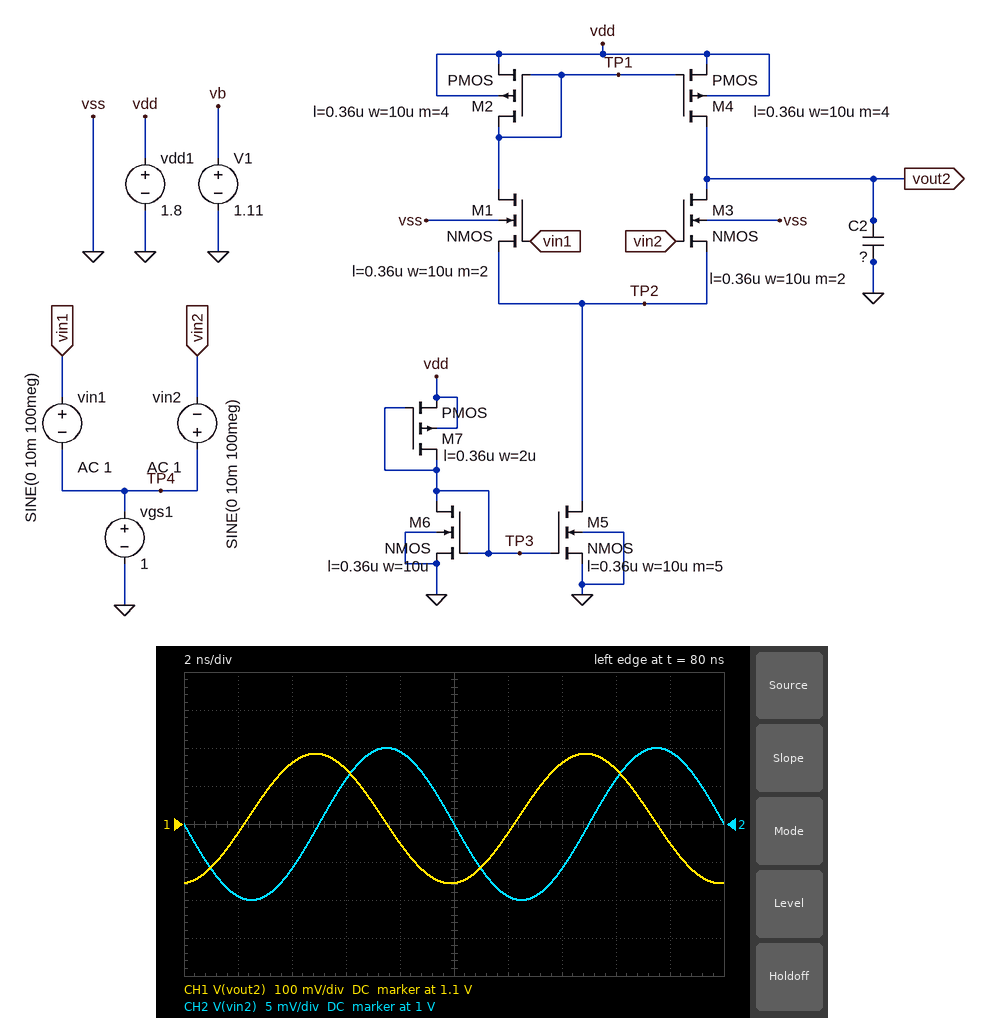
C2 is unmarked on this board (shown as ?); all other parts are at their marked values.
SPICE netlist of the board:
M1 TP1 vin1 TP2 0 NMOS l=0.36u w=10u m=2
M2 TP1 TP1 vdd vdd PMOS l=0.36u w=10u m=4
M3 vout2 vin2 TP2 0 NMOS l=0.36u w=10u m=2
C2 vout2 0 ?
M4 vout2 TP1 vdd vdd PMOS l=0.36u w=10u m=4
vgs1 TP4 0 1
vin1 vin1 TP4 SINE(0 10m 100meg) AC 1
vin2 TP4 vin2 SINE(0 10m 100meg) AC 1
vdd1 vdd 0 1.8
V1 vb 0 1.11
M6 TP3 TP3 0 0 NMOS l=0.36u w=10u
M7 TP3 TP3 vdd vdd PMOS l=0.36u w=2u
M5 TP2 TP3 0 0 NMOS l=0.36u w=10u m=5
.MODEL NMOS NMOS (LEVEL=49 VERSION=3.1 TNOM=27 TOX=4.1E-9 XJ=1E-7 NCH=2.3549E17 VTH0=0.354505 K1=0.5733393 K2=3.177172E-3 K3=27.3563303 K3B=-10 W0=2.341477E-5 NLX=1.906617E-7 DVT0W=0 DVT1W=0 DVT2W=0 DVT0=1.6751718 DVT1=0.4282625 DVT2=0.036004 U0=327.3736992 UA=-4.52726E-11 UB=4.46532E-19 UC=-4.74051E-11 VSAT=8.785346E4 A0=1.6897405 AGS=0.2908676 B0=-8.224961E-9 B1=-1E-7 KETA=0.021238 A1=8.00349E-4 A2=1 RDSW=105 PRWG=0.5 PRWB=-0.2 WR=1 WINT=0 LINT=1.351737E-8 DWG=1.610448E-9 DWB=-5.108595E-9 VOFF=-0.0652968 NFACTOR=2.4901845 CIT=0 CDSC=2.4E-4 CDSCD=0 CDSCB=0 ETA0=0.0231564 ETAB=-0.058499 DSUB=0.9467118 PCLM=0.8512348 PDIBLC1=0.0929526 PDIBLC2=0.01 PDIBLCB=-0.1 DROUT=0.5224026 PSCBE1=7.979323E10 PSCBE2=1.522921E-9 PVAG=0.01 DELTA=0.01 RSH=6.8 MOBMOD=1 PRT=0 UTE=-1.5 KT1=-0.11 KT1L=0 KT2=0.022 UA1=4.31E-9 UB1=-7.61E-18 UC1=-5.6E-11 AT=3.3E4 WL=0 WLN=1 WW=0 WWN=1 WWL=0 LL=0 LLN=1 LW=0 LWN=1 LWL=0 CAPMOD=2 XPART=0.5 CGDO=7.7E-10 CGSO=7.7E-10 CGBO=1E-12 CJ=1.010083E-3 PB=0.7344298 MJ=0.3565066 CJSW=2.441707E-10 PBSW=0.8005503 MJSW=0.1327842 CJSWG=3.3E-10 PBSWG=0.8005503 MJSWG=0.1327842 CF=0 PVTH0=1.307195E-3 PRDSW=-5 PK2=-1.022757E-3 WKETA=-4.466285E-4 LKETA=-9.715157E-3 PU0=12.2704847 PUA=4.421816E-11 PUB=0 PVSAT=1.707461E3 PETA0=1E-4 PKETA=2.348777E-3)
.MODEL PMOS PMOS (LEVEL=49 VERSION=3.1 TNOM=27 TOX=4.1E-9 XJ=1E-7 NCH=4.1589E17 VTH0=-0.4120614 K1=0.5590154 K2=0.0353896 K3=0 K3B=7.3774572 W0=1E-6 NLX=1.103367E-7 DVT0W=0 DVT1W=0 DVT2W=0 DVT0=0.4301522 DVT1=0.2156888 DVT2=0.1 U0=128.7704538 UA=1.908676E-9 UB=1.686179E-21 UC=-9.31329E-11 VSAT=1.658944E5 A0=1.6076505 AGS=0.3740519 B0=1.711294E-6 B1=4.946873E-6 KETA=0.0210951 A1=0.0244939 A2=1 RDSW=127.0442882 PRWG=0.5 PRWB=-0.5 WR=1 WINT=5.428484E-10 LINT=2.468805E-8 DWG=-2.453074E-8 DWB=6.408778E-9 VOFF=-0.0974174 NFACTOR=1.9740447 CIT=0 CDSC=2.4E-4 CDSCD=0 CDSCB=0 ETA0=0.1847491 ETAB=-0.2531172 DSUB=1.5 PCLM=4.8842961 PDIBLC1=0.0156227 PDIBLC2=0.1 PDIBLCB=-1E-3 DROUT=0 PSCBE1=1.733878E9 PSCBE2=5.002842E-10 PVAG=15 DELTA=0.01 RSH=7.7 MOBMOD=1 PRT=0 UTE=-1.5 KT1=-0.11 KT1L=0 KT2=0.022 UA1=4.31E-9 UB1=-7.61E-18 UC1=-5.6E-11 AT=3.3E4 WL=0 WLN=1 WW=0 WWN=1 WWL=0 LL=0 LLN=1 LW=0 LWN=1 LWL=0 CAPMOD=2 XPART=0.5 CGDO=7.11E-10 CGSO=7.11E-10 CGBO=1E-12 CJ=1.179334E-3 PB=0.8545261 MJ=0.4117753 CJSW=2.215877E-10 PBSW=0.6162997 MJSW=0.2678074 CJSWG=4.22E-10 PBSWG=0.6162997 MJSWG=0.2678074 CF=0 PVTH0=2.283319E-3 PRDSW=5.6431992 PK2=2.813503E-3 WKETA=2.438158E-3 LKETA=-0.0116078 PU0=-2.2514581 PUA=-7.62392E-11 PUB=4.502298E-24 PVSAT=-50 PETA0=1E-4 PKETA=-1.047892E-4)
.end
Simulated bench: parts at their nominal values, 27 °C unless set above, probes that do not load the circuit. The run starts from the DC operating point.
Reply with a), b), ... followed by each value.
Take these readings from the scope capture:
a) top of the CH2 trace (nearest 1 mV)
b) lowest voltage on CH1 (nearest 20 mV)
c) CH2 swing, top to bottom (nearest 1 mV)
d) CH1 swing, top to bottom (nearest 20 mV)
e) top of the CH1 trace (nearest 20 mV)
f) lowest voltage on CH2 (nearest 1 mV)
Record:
a) 1.010 V
b) 940 mV
c) 20 mV
d) 340 mV
e) 1.28 V
f) 990 mV
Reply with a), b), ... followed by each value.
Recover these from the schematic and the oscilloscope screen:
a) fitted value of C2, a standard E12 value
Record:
a) 330 fF
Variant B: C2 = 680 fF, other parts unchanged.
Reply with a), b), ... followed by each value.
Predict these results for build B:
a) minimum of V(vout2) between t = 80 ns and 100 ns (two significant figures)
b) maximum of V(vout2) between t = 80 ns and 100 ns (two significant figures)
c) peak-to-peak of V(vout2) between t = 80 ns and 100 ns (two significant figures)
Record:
a) 1.0 V
b) 1.2 V
c) 190 mV
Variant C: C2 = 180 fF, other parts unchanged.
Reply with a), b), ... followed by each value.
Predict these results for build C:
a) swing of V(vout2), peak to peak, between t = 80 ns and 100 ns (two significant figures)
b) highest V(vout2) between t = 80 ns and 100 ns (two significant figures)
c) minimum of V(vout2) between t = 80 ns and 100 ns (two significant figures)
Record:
a) 530 mV
b) 1.4 V
c) 850 mV
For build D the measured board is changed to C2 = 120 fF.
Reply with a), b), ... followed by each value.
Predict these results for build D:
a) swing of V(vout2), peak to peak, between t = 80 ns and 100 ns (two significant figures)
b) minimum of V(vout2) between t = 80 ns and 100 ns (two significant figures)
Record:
a) 670 mV
b) 780 mV
